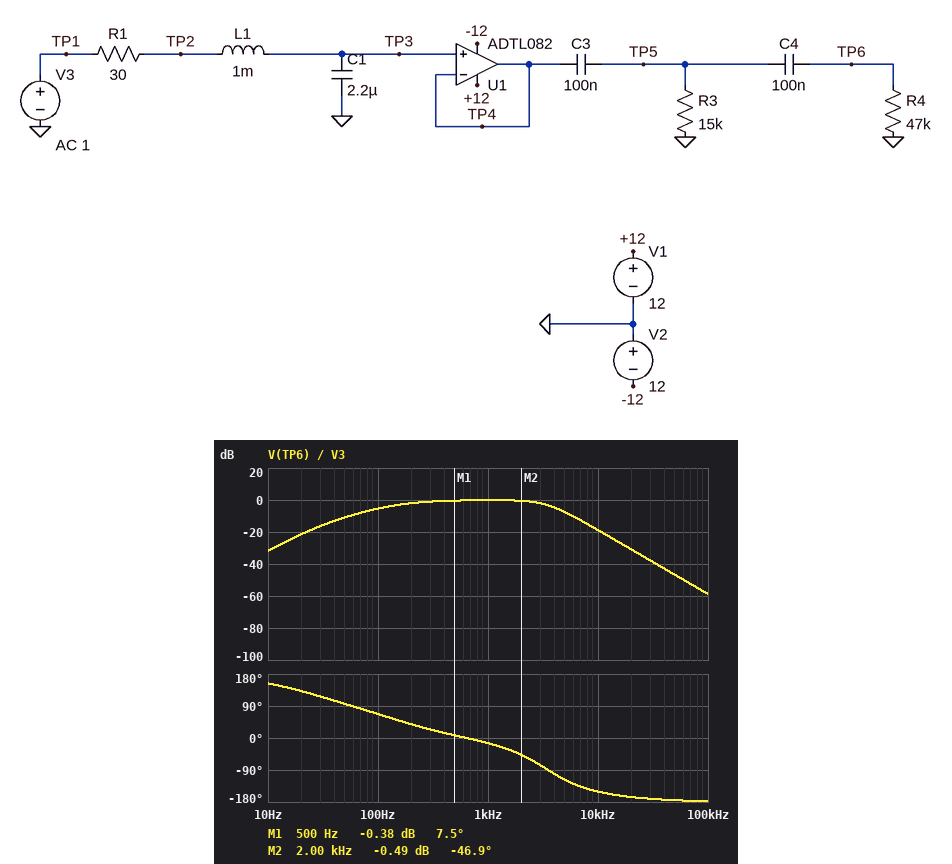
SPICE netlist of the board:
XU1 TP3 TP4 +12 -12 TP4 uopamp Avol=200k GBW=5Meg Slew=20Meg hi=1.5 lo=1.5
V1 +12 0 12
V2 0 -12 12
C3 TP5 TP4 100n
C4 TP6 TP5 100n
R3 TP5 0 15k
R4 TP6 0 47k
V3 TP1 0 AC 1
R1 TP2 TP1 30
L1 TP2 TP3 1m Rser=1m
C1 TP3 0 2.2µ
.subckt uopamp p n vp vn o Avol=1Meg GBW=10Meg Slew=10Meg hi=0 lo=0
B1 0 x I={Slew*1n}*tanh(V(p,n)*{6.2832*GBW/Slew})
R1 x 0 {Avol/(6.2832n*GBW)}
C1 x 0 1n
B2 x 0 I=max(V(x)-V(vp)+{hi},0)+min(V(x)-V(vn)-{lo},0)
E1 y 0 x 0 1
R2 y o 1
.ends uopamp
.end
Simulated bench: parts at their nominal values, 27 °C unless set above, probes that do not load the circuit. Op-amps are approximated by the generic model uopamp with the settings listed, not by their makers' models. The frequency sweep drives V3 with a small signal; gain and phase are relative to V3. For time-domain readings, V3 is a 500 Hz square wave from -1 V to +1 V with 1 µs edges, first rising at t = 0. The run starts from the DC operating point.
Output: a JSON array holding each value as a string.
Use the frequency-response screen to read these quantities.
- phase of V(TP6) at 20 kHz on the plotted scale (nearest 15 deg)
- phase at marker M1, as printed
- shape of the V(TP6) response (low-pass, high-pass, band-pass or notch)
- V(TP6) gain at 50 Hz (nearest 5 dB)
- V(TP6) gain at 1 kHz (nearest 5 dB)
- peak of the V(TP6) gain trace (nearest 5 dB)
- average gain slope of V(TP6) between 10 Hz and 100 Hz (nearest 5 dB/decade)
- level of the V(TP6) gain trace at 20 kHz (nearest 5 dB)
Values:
["-165 deg", "7.5 deg", "band-pass", "-10 dB", "0 dB", "0 dB", "25 dB/decade", "-30 dB"]
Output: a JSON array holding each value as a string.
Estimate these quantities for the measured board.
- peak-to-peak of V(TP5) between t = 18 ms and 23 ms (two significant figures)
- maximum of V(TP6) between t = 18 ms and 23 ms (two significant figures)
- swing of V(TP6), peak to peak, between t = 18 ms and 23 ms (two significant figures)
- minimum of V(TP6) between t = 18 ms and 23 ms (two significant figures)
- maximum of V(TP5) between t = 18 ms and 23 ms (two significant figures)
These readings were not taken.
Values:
["2.7 V", "1.4 V", "2.8 V", "-1.4 V", "1.4 V"]
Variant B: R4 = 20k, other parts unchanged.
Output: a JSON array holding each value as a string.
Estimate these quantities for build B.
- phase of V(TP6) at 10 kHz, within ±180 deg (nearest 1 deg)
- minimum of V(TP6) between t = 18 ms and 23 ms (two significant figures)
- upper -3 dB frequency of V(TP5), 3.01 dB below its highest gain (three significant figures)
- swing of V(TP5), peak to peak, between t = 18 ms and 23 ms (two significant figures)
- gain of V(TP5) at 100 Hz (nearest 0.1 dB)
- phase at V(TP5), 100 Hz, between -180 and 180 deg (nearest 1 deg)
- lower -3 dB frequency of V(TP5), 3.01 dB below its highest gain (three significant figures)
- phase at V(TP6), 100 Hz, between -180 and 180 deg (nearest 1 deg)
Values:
["-150 deg", "-1.5 V", "3.48 kHz", "2.8 V", "-6.4 dB", "46 deg", "196 Hz", "84 deg"]
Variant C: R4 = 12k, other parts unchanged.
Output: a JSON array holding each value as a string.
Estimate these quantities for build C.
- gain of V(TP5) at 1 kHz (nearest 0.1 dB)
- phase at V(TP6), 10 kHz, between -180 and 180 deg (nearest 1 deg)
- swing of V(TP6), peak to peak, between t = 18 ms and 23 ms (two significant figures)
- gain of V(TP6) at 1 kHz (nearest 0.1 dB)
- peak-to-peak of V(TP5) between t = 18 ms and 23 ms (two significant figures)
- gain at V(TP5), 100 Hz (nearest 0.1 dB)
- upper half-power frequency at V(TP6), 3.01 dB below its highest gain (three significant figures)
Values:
["-0.4 dB", "-150 deg", "3.1 V", "-0.5 dB", "2.8 V", "-7.0 dB", "3.53 kHz"]
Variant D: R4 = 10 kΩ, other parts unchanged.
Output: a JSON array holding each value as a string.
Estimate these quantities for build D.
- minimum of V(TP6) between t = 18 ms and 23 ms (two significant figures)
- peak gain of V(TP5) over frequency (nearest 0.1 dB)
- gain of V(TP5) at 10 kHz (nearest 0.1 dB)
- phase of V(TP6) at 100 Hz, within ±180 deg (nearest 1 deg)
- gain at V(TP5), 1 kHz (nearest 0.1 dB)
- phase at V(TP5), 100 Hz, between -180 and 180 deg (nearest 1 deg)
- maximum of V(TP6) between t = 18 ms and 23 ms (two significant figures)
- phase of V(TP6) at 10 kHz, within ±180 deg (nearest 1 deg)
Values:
["-1.6 V", "-0.4 dB", "-18.8 dB", "97 deg", "-0.5 dB", "39 deg", "1.6 V", "-149 deg"]
